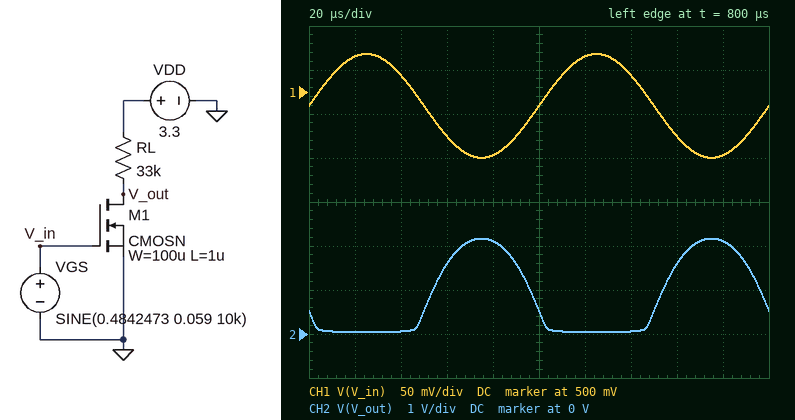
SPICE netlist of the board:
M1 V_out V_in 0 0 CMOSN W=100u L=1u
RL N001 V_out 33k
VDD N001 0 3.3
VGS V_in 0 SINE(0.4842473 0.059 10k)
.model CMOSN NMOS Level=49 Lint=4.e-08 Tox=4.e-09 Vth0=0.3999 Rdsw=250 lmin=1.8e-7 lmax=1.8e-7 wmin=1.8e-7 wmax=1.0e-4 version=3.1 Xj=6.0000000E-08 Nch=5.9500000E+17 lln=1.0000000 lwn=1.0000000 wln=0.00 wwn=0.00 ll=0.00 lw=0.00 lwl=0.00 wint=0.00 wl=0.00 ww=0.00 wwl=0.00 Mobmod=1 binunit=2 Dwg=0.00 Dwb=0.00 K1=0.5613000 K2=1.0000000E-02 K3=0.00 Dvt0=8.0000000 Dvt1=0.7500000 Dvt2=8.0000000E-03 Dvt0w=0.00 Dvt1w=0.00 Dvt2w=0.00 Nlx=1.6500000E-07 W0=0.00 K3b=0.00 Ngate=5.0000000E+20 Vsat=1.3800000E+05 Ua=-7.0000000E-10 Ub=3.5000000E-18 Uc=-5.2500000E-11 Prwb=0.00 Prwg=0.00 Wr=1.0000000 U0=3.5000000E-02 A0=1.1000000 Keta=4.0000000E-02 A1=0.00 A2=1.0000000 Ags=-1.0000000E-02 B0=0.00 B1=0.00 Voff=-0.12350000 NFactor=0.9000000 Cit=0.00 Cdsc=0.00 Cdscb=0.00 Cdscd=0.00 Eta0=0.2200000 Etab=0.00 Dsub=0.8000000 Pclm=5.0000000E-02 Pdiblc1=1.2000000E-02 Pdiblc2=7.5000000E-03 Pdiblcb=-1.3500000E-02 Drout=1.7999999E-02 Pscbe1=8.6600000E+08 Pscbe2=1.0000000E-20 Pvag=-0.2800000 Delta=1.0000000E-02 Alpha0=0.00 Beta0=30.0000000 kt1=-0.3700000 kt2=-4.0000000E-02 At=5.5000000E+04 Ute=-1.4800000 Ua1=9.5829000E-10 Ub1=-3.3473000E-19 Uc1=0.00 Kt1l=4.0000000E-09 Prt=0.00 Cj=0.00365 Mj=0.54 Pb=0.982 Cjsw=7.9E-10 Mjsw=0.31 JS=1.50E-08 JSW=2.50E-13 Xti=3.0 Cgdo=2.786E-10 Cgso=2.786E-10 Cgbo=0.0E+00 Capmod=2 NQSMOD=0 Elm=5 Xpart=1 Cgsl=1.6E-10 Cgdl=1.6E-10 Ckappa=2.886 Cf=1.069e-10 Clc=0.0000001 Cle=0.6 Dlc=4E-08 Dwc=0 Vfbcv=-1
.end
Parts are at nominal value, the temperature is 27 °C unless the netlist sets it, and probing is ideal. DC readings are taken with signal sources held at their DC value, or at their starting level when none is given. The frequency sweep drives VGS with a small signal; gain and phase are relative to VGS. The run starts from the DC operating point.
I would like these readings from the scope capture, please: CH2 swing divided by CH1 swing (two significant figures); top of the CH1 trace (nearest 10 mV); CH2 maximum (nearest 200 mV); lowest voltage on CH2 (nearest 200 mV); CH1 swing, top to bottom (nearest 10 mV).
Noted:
18
540 mV
2.2 V
0 V
120 mV
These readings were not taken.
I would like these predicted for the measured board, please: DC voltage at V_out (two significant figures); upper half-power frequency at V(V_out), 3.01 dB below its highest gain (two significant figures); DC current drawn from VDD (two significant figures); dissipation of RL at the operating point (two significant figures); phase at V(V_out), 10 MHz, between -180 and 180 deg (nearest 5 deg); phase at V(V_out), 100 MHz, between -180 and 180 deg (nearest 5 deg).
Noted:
530 mV
53 MHz
84 µA
230 µW
170 deg
115 deg
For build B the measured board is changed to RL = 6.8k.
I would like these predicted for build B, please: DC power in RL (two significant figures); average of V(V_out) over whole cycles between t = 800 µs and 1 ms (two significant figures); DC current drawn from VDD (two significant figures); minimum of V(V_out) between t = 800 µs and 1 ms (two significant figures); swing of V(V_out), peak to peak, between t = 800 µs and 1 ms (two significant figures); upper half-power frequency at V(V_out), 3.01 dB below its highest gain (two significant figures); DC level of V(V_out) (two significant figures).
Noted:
76 µW
2.5 V
110 µA
1.7 V
1.3 V
250 MHz
2.6 V
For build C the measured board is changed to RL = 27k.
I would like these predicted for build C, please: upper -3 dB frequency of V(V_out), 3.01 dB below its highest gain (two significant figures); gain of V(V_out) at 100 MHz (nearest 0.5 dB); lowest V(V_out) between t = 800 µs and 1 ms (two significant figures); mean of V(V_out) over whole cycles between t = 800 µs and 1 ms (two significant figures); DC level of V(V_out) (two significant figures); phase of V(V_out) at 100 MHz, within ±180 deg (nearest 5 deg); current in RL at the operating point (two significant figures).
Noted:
65 MHz
24.5 dB
52 mV
1.0 V
920 mV
120 deg
88 µA
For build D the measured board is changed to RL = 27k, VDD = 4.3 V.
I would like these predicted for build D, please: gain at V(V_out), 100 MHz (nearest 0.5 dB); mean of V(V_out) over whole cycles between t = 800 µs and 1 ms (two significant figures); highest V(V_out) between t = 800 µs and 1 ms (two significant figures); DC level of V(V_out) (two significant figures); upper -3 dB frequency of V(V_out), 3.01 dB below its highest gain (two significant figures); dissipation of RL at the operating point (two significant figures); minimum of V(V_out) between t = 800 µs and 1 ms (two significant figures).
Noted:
26.0 dB
1.6 V
3.3 V
1.7 V
71 MHz
250 µW
80 mV
